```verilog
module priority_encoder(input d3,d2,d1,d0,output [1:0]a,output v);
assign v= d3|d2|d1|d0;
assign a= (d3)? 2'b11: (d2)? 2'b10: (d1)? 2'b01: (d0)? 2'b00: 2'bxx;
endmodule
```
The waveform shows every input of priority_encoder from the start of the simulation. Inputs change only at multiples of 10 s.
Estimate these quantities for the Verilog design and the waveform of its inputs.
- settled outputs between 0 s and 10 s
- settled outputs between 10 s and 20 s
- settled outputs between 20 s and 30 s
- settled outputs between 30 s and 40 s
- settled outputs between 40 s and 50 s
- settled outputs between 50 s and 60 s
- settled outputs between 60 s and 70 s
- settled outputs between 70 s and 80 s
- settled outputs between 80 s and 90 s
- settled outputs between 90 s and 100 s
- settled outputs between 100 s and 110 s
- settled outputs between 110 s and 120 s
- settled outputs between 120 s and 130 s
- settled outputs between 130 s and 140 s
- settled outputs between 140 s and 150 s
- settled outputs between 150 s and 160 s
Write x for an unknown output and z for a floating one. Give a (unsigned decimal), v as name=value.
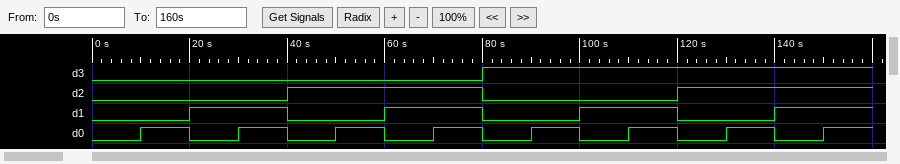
a=x, v=0
a=0, v=1
a=1, v=1
a=1, v=1
a=2, v=1
a=2, v=1
a=2, v=1
a=2, v=1
a=3, v=1
a=3, v=1
a=3, v=1
a=3, v=1
a=3, v=1
a=3, v=1
a=3, v=1
a=3, v=1
